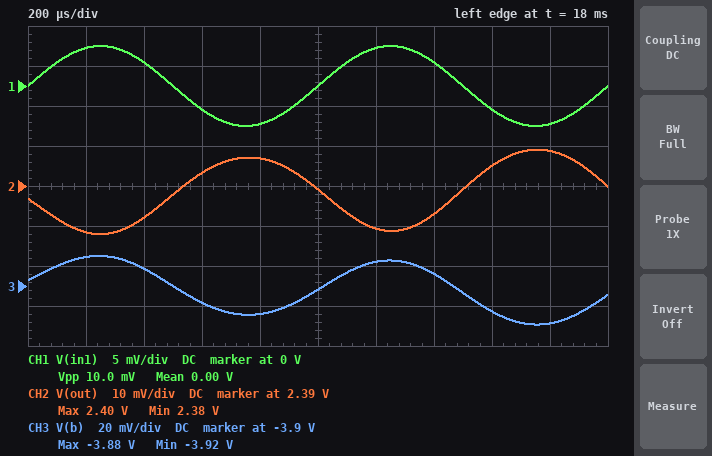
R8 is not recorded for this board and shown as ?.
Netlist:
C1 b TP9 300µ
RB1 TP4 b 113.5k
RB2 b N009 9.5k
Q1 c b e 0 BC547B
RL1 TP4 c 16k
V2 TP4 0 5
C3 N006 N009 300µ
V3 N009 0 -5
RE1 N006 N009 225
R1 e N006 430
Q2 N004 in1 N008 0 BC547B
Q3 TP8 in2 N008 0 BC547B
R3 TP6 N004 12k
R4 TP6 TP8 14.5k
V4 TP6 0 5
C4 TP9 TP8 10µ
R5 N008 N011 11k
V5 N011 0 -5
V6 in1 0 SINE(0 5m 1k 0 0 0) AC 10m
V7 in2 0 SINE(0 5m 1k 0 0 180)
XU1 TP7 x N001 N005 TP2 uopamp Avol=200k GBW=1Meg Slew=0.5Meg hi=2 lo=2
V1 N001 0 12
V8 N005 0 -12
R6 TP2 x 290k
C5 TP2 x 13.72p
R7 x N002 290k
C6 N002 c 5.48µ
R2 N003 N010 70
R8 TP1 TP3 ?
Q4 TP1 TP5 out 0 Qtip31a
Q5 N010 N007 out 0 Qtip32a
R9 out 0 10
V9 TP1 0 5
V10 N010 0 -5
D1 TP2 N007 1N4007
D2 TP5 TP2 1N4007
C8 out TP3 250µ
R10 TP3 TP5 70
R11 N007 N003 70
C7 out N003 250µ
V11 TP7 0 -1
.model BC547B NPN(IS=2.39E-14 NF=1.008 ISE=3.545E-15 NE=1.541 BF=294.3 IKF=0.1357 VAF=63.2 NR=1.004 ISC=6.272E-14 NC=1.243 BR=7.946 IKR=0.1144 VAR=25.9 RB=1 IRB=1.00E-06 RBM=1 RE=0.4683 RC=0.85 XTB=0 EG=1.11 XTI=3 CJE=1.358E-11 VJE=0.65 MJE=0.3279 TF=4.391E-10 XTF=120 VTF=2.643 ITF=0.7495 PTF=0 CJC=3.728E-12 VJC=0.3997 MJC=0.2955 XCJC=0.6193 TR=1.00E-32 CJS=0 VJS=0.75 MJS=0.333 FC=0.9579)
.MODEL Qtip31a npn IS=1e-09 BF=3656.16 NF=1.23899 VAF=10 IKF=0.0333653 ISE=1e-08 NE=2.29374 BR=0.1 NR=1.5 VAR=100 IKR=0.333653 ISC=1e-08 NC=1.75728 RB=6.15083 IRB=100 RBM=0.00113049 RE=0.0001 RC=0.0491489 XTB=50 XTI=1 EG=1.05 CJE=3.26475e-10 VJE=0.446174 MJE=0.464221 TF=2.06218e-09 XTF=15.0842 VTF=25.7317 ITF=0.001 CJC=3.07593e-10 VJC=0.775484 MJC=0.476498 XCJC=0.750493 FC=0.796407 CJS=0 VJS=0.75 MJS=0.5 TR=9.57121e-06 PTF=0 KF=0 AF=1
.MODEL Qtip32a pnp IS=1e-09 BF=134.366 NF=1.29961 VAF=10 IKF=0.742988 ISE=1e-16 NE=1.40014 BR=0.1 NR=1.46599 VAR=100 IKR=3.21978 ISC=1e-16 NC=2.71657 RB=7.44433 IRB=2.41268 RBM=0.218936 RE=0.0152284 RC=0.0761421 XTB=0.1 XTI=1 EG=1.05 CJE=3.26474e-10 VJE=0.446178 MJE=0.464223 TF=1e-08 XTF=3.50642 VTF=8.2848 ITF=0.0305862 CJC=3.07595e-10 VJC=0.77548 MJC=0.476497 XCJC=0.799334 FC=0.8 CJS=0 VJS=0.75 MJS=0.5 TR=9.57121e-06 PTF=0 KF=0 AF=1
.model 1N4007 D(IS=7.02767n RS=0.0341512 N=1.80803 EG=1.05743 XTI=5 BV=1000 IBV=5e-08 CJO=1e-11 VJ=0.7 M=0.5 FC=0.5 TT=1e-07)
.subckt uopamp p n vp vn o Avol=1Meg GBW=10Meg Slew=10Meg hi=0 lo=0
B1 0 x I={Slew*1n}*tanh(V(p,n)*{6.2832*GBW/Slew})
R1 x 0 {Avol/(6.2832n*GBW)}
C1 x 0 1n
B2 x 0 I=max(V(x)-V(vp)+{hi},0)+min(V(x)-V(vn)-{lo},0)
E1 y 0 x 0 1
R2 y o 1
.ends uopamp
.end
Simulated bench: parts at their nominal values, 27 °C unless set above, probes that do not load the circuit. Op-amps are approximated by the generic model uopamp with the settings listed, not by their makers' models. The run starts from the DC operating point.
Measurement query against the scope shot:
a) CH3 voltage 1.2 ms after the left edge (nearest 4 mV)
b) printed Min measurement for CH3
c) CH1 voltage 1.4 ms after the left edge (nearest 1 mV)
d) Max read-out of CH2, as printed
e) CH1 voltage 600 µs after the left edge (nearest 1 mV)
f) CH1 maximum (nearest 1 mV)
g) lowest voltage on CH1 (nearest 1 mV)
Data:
-3.888 V
-3.92 V
3 mV
2.40 V
-3 mV
5 mV
-5 mV
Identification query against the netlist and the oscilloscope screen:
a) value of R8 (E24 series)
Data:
180 Ω
